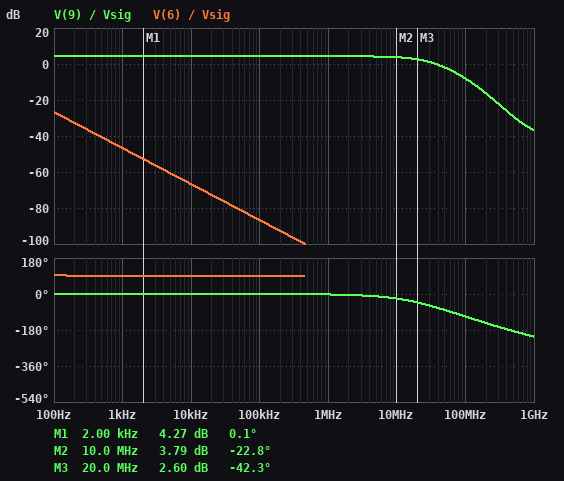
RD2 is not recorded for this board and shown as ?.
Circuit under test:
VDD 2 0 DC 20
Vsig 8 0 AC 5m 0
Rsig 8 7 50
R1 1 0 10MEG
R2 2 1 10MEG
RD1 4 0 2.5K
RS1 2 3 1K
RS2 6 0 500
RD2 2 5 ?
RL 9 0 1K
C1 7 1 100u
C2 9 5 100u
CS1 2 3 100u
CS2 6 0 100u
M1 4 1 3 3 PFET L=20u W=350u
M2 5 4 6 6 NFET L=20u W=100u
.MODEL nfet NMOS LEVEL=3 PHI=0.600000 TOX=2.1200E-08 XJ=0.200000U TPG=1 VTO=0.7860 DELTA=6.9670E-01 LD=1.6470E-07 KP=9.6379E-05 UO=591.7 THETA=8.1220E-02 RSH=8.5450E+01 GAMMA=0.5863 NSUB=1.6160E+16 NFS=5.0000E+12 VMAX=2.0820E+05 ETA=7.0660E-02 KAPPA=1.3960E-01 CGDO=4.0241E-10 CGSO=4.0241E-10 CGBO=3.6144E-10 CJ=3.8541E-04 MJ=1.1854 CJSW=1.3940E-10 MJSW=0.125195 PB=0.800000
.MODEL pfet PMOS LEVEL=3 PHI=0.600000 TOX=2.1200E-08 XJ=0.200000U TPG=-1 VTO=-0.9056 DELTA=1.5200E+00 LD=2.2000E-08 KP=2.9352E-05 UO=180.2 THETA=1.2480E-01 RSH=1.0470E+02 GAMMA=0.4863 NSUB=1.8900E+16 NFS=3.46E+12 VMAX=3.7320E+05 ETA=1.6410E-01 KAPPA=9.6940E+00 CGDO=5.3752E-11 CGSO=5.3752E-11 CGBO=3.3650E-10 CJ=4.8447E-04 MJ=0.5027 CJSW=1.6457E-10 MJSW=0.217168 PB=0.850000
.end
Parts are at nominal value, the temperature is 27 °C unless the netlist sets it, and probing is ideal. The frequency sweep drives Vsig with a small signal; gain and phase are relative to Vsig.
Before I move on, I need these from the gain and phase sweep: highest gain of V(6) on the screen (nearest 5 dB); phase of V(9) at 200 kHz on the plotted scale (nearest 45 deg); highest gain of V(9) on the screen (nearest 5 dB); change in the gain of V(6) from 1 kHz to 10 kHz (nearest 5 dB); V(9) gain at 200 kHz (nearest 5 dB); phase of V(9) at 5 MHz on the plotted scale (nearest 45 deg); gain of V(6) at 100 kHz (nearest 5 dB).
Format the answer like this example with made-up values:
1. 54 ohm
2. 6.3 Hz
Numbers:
1. -25 dB
2. 0 deg
3. 5 dB
4. -20 dB
5. 5 dB
6. 0 deg
7. -85 dB
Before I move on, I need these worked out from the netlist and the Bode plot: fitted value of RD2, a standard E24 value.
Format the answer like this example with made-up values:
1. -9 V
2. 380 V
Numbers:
1. 1.3 kΩ
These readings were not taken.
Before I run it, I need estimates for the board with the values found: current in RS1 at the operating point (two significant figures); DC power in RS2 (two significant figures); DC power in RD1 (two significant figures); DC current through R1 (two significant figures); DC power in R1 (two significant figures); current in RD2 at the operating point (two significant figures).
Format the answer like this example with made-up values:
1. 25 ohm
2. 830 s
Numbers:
1. 3.6 mA
2. 9.2 mW
3. 32 mW
4. 1.0 µA
5. 10 µW
6. 4.3 mA
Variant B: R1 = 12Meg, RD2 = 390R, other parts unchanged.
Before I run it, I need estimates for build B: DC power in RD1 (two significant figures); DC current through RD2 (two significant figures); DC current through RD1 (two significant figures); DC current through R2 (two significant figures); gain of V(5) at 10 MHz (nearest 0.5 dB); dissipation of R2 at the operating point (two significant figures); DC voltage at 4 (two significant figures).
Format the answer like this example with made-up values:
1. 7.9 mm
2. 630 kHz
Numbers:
1. 24 mW
2. 3.5 mA
3. 3.1 mA
4. 910 nA
5. -3.0 dB
6. 8.3 µW
7. 7.8 V
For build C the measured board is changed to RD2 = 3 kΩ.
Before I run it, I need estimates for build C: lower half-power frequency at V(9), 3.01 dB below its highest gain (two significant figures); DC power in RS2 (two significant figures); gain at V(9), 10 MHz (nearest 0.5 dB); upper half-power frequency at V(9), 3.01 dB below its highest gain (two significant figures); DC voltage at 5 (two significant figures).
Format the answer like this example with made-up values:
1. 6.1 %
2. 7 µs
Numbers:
1. 4.4 Hz
2. 9.1 mW
3. 4.5 dB
4. 23 MHz
5. 7.2 V
